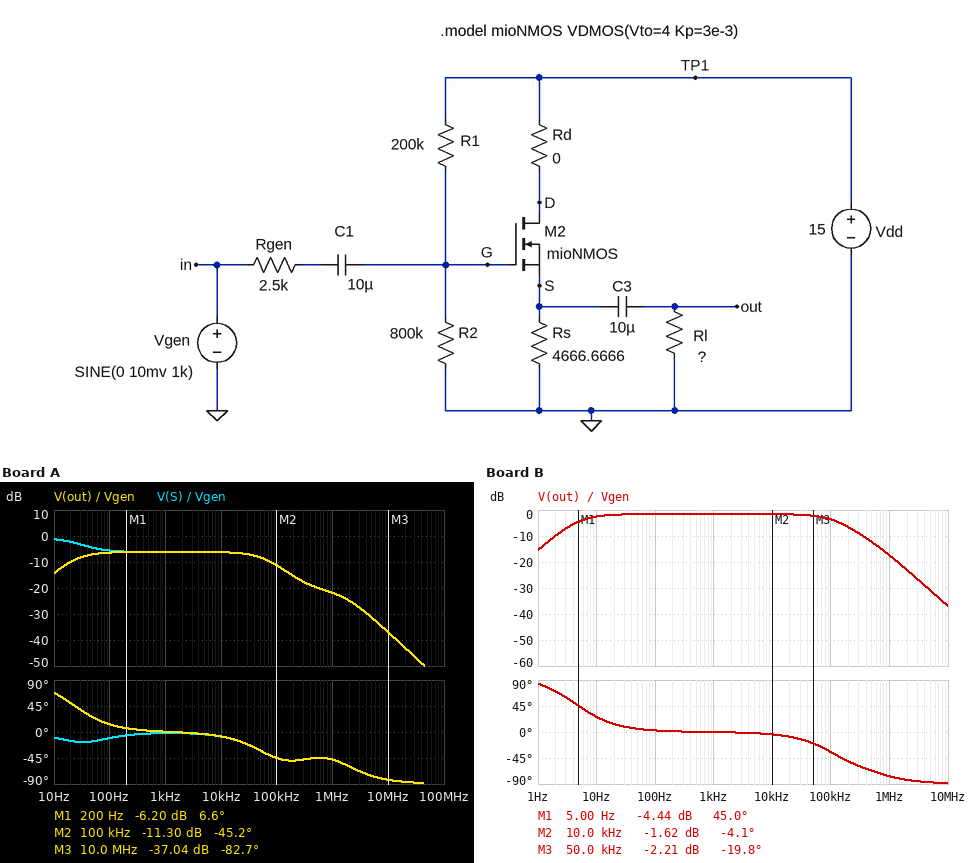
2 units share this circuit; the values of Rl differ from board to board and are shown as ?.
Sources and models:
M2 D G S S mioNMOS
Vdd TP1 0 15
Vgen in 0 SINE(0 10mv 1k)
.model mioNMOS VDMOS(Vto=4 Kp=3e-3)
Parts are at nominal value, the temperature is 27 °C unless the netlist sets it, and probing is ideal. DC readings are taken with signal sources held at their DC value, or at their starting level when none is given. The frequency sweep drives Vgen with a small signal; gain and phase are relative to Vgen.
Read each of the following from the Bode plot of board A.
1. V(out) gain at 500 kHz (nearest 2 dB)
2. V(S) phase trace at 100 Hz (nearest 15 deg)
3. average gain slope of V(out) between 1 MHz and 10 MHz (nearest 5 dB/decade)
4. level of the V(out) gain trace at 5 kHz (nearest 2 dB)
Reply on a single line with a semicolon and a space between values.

-20 dB; -15 deg; -15 dB/decade; -6 dB
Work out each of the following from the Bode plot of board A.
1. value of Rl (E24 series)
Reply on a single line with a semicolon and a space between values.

360 Ω
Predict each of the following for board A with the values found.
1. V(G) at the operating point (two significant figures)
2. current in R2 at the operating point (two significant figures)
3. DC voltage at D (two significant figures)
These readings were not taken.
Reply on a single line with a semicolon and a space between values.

12 V; 15 µA; 15 V
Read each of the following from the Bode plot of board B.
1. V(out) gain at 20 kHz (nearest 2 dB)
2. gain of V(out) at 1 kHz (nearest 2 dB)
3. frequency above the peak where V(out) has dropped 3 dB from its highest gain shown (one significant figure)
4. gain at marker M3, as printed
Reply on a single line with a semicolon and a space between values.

-2 dB; -2 dB; 100 kHz; -2.21 dB
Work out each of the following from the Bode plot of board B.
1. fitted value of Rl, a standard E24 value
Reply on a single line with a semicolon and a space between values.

3 kΩ
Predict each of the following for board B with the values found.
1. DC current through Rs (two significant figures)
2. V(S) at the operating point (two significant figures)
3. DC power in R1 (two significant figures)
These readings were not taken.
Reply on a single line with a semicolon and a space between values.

1.5 mA; 7.0 V; 45 µW
